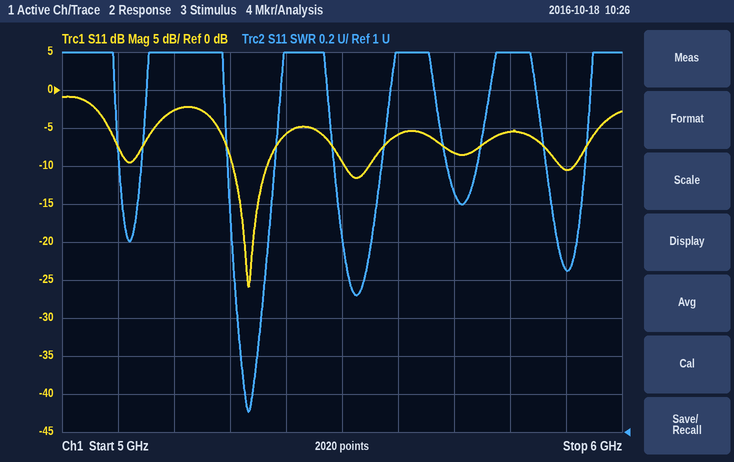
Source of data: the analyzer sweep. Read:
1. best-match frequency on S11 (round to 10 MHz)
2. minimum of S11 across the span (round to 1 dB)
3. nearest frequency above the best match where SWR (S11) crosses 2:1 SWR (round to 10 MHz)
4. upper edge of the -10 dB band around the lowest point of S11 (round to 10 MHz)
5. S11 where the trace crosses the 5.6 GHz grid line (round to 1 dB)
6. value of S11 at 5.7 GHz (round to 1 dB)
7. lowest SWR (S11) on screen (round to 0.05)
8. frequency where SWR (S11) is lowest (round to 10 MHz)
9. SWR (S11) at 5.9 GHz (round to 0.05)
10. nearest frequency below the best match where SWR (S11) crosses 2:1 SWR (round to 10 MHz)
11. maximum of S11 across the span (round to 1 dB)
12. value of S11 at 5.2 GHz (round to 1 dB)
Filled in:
5.33 GHz
-26 dB
5.37 GHz
5.37 GHz
-6 dB
-8 dB
1.10
5.33 GHz
1.85
5.30 GHz
-1 dB
-3 dB
